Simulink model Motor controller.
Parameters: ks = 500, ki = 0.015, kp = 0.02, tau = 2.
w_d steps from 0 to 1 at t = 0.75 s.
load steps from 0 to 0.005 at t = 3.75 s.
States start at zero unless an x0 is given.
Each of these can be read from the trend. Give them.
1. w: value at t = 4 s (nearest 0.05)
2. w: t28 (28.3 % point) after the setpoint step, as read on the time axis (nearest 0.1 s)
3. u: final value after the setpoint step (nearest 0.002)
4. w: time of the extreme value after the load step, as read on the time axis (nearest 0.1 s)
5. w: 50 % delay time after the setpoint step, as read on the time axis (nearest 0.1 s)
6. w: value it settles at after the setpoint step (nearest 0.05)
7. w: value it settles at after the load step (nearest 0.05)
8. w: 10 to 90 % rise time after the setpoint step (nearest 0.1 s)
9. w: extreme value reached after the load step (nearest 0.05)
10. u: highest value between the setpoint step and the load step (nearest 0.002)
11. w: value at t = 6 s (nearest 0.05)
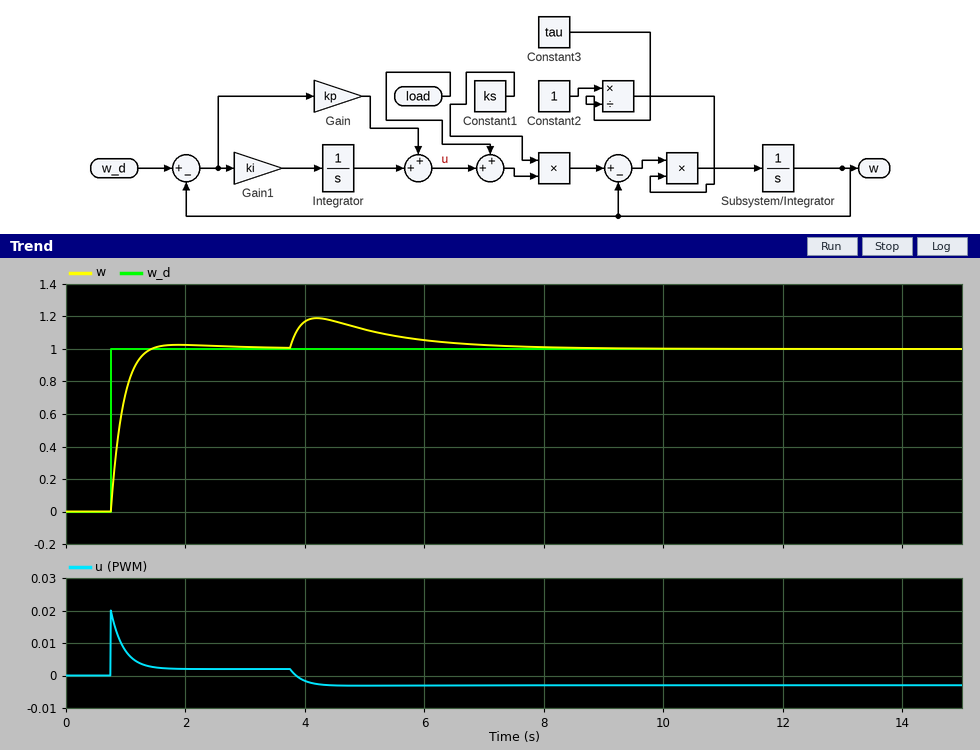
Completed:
1.15
0.8 s
0.002
4.2 s
0.9 s
1.00
1.00
0.4 s
1.20
0.020
1.05
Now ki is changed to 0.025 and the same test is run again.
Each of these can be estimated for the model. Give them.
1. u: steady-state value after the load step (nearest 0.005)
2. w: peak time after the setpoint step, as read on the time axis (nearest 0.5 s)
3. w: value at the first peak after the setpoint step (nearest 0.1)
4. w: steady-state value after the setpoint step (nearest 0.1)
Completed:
-0.005
1.5 s
1.1
1.0
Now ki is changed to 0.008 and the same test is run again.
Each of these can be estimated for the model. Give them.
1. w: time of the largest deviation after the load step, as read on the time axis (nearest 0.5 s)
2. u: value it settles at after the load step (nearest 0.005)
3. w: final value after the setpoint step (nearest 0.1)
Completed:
4.5 s
-0.005
1.0
